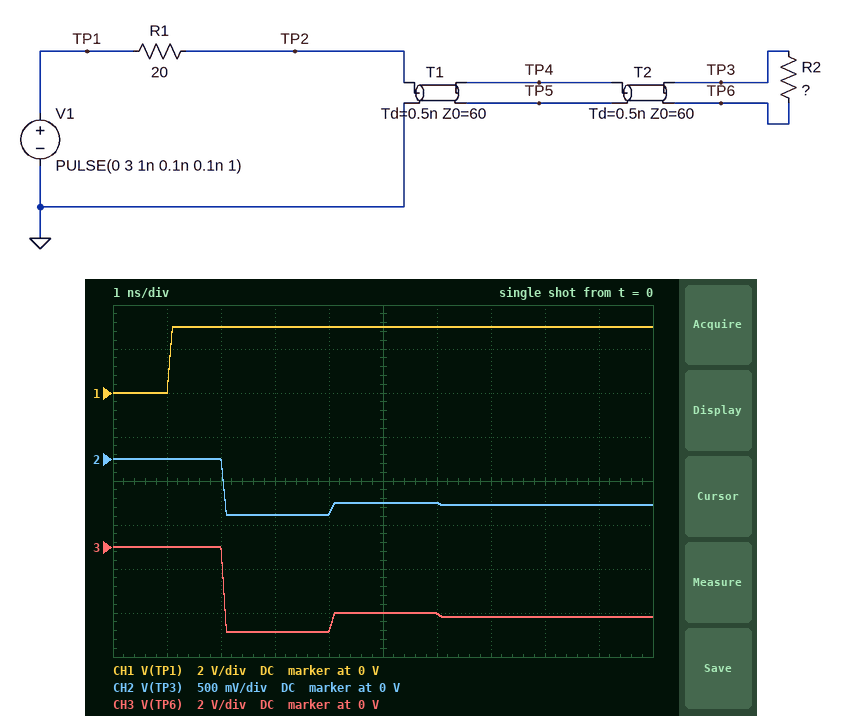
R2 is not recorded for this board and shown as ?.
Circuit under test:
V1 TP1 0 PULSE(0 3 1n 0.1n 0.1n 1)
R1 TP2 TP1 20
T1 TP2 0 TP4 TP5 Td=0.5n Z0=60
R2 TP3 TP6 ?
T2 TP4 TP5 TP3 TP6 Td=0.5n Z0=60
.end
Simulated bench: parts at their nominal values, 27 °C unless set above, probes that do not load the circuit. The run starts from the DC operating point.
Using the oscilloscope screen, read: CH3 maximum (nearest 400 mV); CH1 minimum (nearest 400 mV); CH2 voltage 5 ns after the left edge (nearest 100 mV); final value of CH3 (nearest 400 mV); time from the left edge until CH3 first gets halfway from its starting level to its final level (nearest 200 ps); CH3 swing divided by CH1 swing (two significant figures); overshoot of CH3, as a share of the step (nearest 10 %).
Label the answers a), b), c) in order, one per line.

a) 0 V
b) 0 V
c) -500 mV
d) -3.2 V
e) 2.0 ns
f) 1.3
g) 20 %
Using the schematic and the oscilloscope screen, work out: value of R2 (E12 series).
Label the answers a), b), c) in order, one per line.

a) 150 Ω
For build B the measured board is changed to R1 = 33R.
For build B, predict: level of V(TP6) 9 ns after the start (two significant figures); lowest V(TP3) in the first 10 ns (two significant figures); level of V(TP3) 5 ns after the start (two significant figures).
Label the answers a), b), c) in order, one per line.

a) -2.9 V
b) -540 mV
c) -480 mV
